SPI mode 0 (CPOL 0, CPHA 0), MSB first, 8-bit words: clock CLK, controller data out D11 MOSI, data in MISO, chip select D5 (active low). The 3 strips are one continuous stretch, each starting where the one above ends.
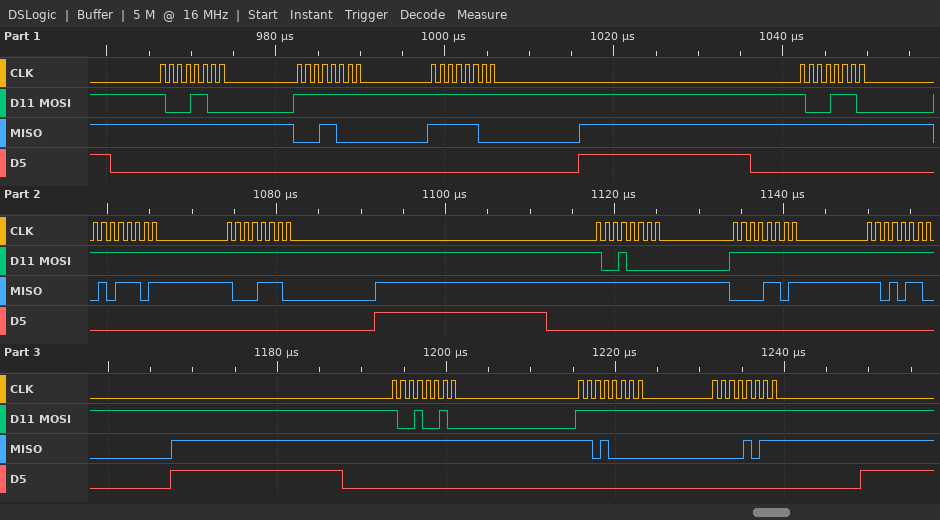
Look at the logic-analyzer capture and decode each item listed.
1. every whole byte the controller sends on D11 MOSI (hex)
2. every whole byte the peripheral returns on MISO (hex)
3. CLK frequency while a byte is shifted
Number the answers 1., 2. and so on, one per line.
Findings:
1. 8C FF FF 8E FF FF 90 FF FF 92 FF FF
2. FF 18 FC FF 5D 8E FF 0D D6 FF D0 0B
3. 1 MHz
